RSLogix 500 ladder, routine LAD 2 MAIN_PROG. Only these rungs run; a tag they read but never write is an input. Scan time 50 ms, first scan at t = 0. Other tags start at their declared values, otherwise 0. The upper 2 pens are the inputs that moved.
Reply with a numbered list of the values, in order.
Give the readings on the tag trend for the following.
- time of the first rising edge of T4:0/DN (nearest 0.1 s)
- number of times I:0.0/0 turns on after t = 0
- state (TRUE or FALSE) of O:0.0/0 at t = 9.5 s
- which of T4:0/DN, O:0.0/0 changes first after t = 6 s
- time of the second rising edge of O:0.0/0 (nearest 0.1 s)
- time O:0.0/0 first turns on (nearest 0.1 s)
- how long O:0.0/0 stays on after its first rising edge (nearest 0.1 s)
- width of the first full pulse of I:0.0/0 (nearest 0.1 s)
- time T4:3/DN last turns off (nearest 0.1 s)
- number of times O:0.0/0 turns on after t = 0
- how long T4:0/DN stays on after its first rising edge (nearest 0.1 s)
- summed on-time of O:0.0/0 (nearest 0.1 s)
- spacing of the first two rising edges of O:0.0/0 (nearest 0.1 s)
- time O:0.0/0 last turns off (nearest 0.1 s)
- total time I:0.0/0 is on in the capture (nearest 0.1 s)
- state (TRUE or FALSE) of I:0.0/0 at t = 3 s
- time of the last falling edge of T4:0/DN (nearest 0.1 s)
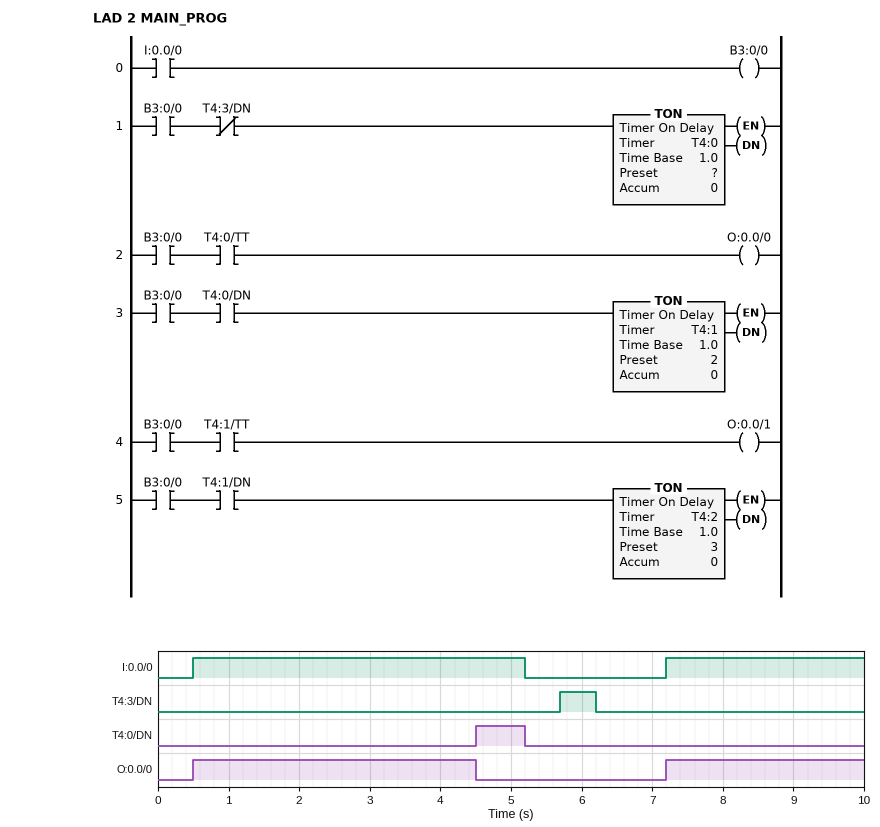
1. 4.5 s
2. 2
3. TRUE
4. O:0.0/0
5. 7.2 s
6. 0.5 s
7. 4.0 s
8. 4.7 s
9. 6.2 s
10. 2
11. 0.7 s
12. 6.8 s
13. 6.7 s
14. 4.5 s
15. 7.5 s
16. TRUE
17. 5.2 s
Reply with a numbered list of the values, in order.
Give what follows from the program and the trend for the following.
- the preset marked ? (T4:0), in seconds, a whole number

1. 4 s
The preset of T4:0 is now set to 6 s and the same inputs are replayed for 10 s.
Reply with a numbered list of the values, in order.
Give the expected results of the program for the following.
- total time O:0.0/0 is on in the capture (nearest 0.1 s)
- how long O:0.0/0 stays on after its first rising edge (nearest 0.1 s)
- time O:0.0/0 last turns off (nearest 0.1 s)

1. 7.5 s
2. 4.7 s
3. 5.2 s
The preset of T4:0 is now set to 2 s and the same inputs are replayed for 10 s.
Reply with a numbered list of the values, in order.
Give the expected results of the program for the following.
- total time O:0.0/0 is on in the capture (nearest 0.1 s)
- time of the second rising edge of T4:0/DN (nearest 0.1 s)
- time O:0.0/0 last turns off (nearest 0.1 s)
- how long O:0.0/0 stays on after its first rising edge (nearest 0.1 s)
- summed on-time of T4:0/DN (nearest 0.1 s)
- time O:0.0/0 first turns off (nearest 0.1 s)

1. 4.0 s
2. 9.2 s
3. 9.2 s
4. 2.0 s
5. 3.5 s
6. 2.5 s
